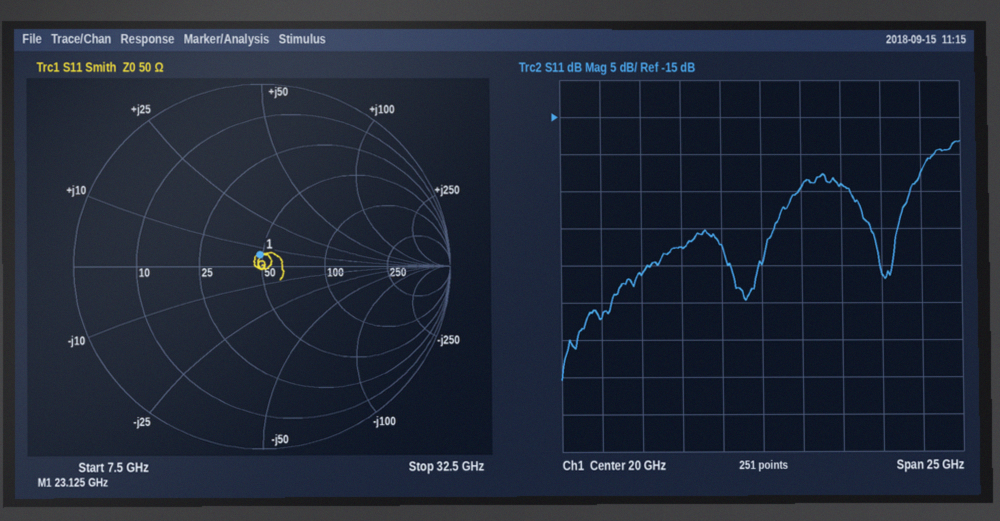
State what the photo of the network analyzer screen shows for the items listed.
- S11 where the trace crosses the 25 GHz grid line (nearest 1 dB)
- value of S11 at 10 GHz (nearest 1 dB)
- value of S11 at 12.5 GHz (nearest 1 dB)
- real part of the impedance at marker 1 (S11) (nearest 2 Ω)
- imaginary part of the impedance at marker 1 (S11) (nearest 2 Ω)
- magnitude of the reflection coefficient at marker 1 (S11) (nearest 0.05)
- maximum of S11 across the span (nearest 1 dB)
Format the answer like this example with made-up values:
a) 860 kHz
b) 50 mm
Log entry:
a) -24 dB
b) -42 dB
c) -36 dB
d) 48 Ω
e) +6 Ω
f) 0.05
g) -18 dB
